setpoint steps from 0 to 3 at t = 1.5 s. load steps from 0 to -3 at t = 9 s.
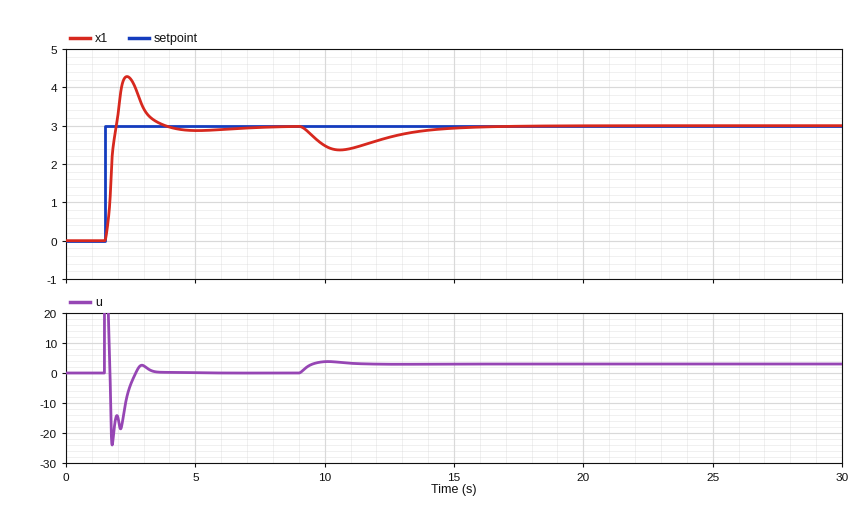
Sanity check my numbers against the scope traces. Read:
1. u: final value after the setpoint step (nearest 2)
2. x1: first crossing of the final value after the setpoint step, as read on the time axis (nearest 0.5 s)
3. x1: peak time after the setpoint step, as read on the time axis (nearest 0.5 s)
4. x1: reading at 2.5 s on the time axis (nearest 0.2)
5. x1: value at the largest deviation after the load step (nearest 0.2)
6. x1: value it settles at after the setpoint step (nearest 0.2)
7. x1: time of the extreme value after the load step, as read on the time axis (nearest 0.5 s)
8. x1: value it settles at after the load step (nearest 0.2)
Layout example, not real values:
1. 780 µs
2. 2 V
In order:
1. 0
2. 2.0 s
3. 2.5 s
4. 4.2
5. 2.4
6. 3.0
7. 10.5 s
8. 3.0
